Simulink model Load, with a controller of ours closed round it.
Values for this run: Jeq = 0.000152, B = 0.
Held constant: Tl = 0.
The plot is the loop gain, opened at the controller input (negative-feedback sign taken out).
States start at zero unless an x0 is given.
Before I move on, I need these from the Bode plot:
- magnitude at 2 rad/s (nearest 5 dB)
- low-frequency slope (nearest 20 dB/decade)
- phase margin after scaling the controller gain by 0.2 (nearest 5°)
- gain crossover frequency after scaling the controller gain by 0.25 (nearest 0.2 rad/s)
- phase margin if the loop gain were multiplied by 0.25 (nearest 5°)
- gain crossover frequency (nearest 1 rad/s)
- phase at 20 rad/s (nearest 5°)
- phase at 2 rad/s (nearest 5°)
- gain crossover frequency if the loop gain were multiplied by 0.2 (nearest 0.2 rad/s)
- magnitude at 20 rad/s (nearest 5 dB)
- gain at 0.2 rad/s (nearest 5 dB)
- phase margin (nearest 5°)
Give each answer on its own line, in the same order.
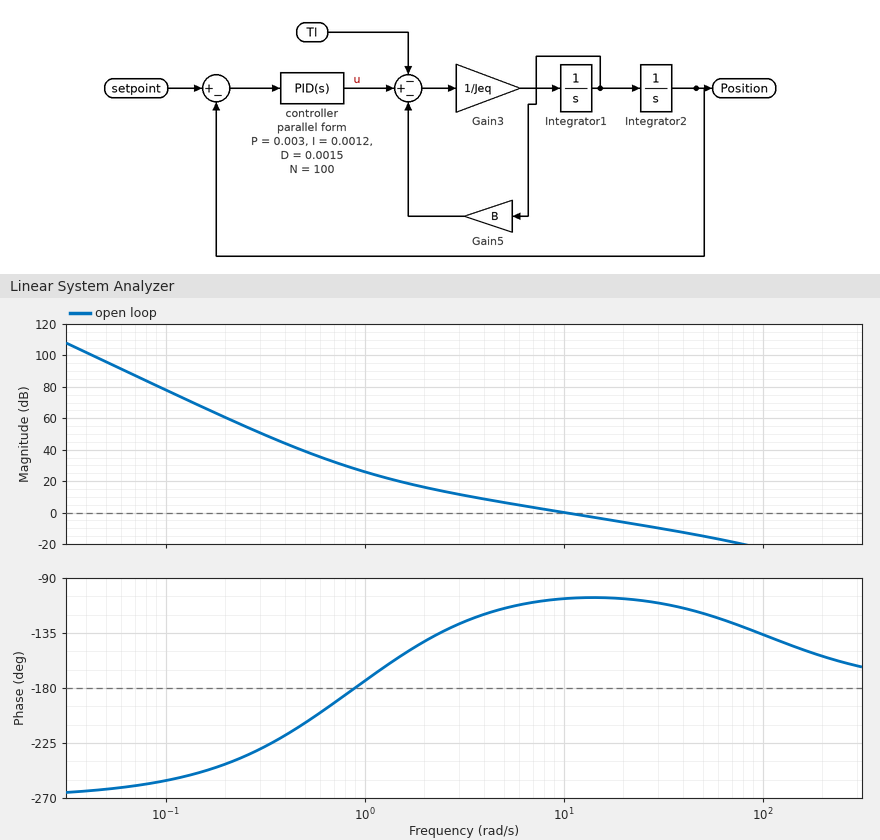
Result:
15 dB
-60 dB/decade
45°
2.8 rad/s
50°
10 rad/s
-105°
-140°
2.4 rad/s
-5 dB
60 dB
75°
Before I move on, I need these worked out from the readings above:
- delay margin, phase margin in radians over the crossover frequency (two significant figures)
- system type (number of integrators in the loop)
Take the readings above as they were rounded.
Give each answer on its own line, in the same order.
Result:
0.13 s
3
